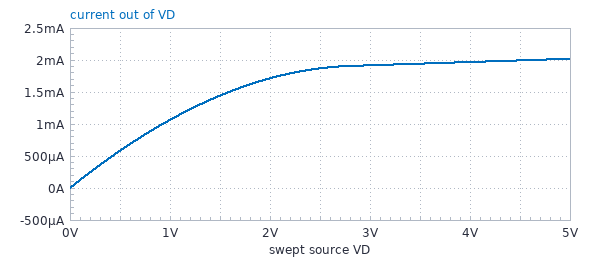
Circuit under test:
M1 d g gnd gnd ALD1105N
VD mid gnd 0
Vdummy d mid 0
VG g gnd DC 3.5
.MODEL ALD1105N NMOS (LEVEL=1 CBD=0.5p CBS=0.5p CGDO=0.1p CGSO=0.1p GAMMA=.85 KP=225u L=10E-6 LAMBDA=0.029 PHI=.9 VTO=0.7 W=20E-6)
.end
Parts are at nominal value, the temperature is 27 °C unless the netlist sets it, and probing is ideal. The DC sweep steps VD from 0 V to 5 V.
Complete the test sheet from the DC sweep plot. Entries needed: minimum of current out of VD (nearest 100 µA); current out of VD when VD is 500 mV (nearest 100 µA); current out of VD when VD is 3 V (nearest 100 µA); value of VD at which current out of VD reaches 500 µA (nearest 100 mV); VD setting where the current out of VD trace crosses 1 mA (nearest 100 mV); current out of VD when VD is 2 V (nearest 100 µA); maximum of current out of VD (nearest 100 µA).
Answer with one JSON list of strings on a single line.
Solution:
["0 A", "600 µA", "1.9 mA", "400 mV", "900 mV", "1.7 mA", "2.0 mA"]
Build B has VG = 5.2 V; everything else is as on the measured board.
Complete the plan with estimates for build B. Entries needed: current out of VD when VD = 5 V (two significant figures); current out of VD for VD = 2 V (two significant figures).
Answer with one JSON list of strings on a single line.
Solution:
["5.2 mA", "3.3 mA"]
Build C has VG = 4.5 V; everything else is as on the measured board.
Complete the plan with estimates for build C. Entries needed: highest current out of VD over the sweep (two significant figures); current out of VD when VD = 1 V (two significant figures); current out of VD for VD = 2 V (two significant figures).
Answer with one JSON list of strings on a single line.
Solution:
["3.7 mA", "1.5 mA", "2.7 mA"]
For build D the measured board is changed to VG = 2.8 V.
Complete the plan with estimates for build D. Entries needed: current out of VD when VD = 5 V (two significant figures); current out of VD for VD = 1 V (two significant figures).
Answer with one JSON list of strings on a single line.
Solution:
["1.1 mA", "740 µA"]
